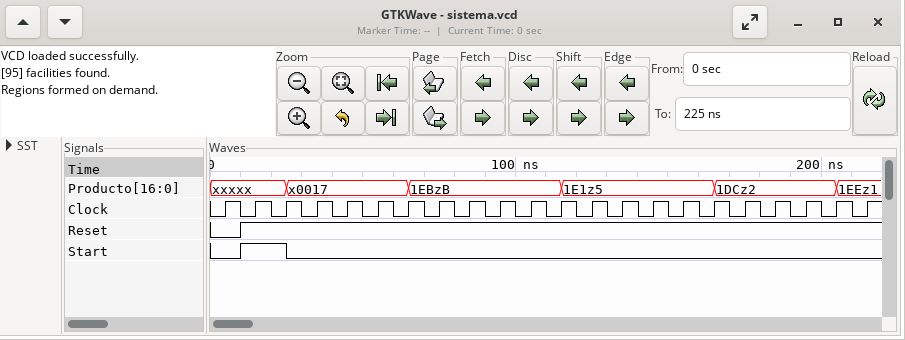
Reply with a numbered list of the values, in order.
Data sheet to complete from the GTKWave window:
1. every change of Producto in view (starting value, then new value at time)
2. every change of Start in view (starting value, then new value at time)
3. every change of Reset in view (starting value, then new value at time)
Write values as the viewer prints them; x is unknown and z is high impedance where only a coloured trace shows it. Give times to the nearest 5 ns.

1. xxxxx, x0017 at 25 ns, 1EBzB at 65 ns, 1E1z5 at 115 ns, 1DCz2 at 165 ns, 1EEz1 at 205 ns
2. 0, 1 at 10 ns, 0 at 25 ns
3. 0, 1 at 10 ns
